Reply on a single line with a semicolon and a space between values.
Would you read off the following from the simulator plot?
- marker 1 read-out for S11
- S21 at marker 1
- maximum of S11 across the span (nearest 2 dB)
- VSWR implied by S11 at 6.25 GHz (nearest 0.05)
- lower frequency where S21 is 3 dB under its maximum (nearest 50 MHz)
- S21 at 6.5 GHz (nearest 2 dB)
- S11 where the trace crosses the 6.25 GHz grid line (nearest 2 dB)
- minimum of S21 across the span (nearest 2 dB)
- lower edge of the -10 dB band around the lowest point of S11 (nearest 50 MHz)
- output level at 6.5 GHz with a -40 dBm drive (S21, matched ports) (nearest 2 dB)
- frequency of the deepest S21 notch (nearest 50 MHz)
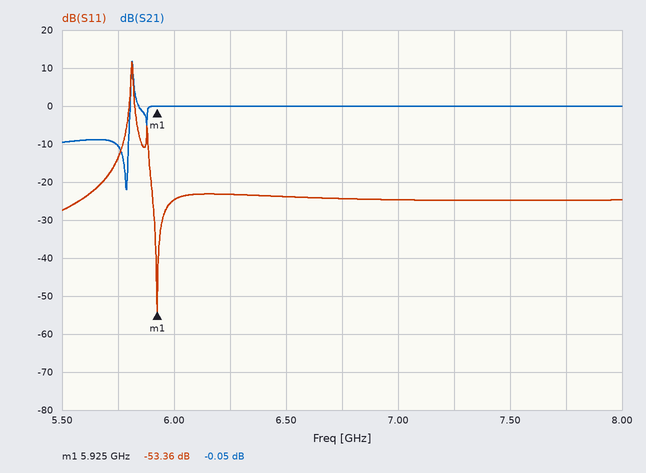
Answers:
-53.36 dB; -0.05 dB; 12 dB; 1.15; 5.80 GHz; 0 dB; -24 dB; -22 dB; 5.90 GHz; -40 dBm; 5.80 GHz
